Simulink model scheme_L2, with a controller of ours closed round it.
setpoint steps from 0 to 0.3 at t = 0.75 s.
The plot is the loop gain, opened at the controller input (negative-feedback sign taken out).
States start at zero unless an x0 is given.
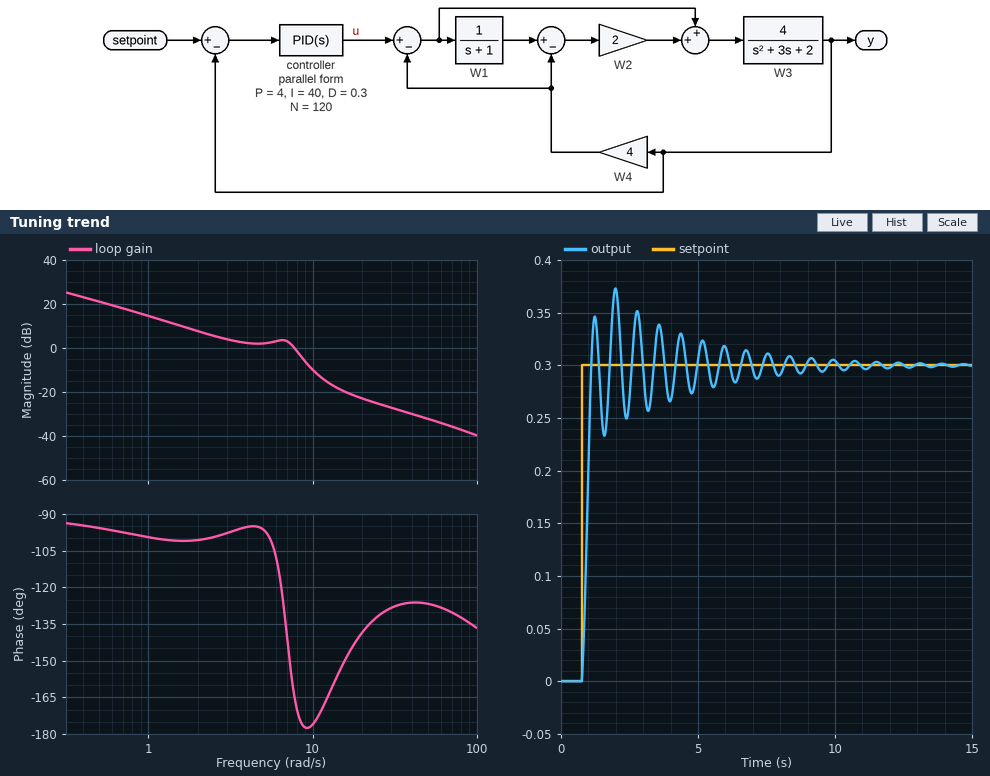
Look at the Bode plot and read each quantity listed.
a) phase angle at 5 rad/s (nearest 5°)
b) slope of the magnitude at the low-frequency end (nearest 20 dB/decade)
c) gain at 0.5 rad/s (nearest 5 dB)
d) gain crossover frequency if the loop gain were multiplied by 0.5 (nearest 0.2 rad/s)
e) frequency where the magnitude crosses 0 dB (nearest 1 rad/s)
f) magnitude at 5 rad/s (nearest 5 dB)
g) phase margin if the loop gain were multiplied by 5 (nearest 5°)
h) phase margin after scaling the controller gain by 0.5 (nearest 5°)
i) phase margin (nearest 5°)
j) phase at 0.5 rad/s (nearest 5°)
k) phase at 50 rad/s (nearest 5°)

-95°
-20 dB/decade
20 dB
2.4 rad/s
8 rad/s
0 dB
10°
80°
15°
-95°
-125°
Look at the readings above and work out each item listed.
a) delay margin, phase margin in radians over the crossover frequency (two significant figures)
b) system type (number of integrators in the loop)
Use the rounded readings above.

0.033 s
1
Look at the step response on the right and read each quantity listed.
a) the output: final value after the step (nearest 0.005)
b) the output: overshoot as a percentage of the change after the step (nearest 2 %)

0.300
24 %
